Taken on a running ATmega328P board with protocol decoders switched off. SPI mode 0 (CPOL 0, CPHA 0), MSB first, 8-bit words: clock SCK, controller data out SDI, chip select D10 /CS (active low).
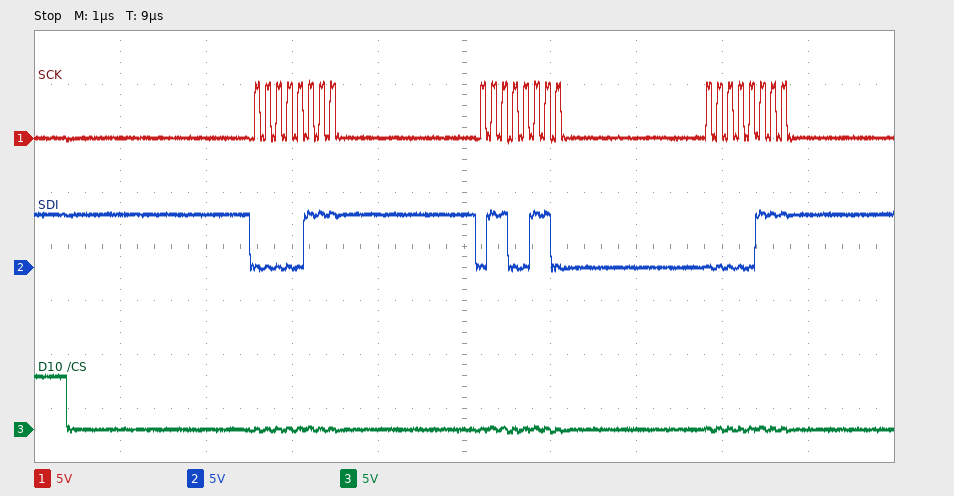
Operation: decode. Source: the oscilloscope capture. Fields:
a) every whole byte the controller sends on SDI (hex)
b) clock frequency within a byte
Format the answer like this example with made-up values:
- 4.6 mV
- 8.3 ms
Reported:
- 07 66 07
- 8 MHz
